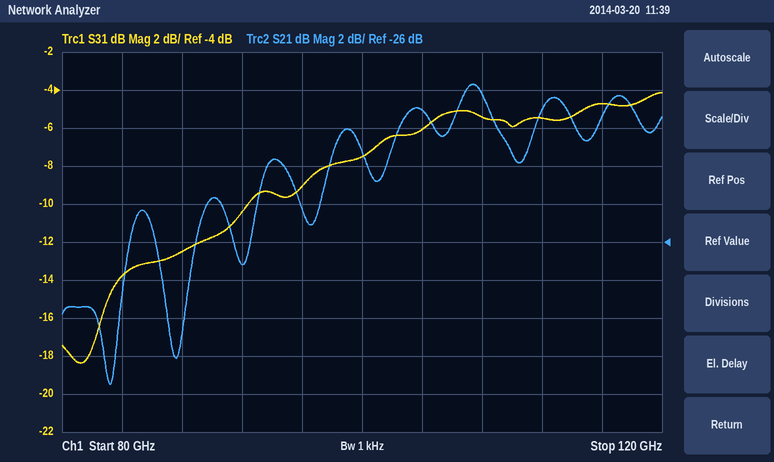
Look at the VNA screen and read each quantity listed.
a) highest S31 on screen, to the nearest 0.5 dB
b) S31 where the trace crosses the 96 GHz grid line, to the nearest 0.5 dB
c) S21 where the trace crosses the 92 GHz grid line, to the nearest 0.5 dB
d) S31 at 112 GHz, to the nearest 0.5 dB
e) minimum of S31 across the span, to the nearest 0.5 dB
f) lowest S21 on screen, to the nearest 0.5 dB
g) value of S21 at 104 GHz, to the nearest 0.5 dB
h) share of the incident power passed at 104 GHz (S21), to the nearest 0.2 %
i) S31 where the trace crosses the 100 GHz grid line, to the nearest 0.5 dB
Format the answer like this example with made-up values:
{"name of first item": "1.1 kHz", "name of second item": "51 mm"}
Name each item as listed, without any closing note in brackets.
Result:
{"highest S31 on screen, to the nearest 0.5 dB": "-4.0 dB", "S31 where the trace crosses the 96 GHz grid line, to the nearest 0.5 dB": "-9.0 dB", "S21 where the trace crosses the 92 GHz grid line, to the nearest 0.5 dB": "-27.0 dB", "S31 at 112 GHz, to the nearest 0.5 dB": "-5.5 dB", "minimum of S31 across the span, to the nearest 0.5 dB": "-18.5 dB", "lowest S21 on screen, to the nearest 0.5 dB": "-33.5 dB", "value of S21 at 104 GHz, to the nearest 0.5 dB": "-19.0 dB", "share of the incident power passed at 104 GHz (S21), to the nearest 0.2 %": "1.2 %", "S31 where the trace crosses the 100 GHz grid line, to the nearest 0.5 dB": "-7.5 dB"}
